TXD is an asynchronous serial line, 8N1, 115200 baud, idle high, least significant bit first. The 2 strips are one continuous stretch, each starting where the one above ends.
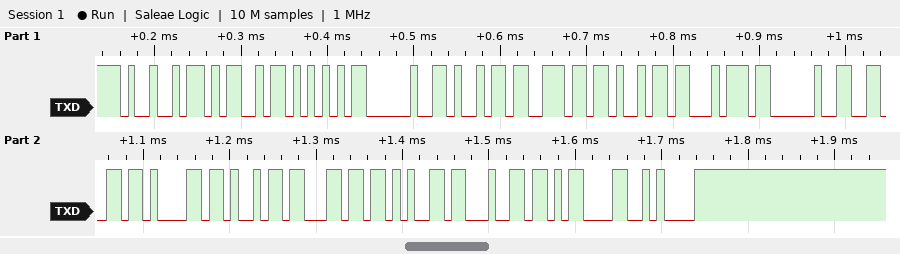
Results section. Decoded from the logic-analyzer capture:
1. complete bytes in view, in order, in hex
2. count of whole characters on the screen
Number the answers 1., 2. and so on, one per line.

1. 0x49 0x4D 0x55 0x20 0x69 0x6E 0x69 0x74 0x20 0x66 0x61 0x69 0x6C 0x65 0x64 0x0D 0x0A
2. 17
